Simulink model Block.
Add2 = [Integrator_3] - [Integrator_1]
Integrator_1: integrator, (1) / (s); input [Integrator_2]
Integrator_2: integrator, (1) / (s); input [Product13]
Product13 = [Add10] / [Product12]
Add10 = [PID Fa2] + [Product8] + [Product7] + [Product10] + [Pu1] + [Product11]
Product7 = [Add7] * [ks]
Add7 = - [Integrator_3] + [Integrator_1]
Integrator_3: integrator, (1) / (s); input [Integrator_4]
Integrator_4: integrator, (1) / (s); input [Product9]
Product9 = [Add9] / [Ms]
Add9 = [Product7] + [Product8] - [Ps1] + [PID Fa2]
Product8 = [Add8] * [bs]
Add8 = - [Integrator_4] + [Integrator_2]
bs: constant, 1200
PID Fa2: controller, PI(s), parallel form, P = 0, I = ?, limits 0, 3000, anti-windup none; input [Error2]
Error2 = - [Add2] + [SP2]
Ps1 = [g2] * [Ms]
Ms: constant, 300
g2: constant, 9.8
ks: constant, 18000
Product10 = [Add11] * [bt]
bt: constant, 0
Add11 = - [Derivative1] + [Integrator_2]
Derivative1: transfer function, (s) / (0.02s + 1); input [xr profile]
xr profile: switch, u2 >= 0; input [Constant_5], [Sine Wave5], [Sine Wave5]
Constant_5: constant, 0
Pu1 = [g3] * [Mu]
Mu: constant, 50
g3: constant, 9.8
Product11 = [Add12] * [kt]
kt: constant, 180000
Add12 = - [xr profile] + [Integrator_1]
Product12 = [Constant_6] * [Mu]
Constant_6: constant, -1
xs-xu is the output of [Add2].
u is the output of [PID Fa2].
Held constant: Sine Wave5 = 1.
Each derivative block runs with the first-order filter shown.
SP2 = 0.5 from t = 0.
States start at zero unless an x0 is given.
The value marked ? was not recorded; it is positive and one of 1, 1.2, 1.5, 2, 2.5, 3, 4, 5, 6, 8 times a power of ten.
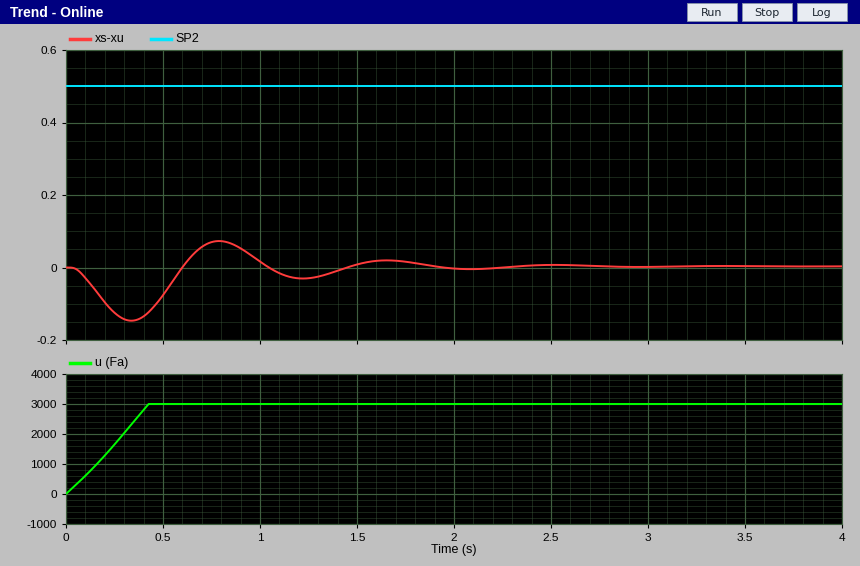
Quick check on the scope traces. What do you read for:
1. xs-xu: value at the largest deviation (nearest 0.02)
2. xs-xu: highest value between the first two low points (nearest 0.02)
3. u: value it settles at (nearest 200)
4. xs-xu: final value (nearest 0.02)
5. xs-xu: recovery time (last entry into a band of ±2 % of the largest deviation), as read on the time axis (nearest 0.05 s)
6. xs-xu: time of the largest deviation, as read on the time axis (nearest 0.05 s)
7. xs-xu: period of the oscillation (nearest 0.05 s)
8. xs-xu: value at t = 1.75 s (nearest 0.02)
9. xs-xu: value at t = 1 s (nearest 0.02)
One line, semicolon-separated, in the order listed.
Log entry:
-0.14; 0.08; 3000; 0.00; 2.60 s; 0.35 s; 0.90 s; 0.02; 0.02
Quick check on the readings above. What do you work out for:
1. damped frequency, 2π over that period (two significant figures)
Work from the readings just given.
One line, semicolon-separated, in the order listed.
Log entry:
7.0 rad/s
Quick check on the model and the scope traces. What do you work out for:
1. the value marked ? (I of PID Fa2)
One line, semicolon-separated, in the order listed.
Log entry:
12000
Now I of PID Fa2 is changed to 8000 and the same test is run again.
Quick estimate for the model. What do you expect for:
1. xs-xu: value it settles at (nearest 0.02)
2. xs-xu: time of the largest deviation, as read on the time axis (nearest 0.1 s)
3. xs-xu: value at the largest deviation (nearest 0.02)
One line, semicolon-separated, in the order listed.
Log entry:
0.00; 0.4 s; -0.18
